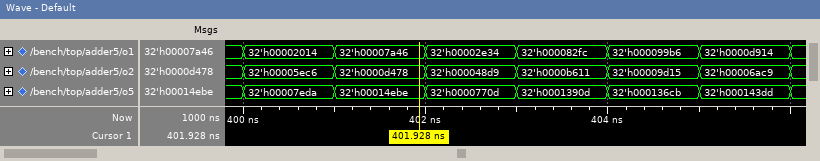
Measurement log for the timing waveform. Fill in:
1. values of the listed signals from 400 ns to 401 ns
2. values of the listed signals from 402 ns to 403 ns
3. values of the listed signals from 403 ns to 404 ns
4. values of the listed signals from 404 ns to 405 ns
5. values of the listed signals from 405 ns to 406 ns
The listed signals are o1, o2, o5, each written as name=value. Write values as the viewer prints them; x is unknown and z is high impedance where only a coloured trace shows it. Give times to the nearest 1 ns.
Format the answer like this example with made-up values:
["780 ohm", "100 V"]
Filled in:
["o1=32'h00002014, o2=32'h00005ec6, o5=32'h00007eda", "o1=32'h00002e34, o2=32'h000048d9, o5=32'h0000770d", "o1=32'h000082fc, o2=32'h0000b611, o5=32'h0001390d", "o1=32'h000099b6, o2=32'h00009d15, o5=32'h000136cb", "o1=32'h0000d914, o2=32'h00006ac9, o5=32'h000143dd"]
